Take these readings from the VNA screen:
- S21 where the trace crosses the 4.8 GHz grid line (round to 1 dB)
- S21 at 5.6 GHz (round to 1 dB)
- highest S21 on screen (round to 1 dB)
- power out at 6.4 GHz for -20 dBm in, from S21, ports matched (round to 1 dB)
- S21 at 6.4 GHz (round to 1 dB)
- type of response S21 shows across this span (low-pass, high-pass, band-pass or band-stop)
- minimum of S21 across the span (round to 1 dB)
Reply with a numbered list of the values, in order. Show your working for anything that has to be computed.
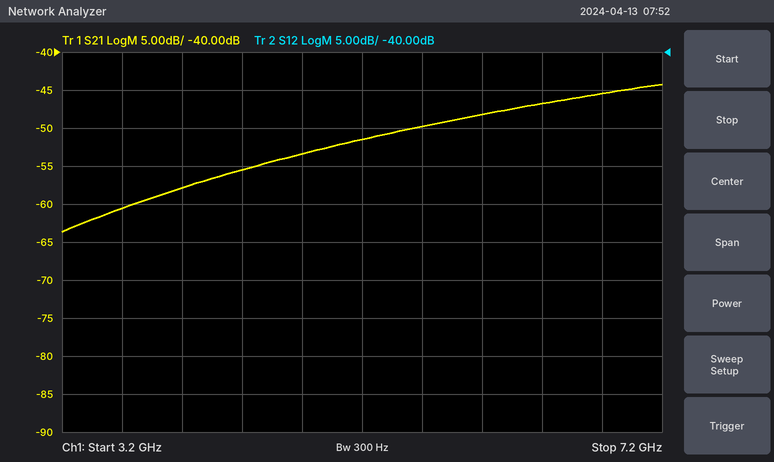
1. -53 dB
2. -50 dB
3. -44 dB
4. -20 dBm + (-47 dB) = -67 dBm
5. -47 dB
6. high-pass
7. -64 dB
